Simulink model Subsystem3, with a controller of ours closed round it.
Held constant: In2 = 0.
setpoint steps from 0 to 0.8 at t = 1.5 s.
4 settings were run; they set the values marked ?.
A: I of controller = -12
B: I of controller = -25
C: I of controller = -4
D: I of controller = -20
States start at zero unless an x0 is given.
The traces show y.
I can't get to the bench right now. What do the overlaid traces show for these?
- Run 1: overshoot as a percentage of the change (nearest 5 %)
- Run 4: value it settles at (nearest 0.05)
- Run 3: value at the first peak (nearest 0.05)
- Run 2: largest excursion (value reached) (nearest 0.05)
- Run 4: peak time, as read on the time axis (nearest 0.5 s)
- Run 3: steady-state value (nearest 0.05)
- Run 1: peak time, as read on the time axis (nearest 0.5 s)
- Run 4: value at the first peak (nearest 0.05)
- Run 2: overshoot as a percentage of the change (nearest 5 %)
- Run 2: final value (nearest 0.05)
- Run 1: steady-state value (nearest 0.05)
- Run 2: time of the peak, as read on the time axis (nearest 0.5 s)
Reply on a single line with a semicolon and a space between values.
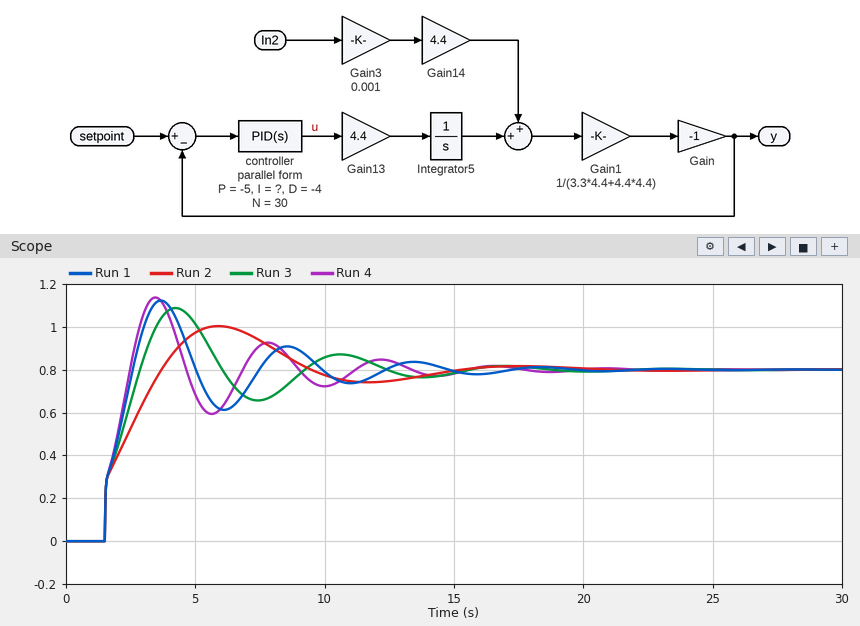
40 %; 0.80; 1.10; 1.00; 3.5 s; 0.80; 3.5 s; 1.15; 25 %; 0.80; 0.80; 6.0 s
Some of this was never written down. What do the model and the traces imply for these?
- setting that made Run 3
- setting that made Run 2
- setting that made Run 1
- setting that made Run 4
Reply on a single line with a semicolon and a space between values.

A; C; D; B
